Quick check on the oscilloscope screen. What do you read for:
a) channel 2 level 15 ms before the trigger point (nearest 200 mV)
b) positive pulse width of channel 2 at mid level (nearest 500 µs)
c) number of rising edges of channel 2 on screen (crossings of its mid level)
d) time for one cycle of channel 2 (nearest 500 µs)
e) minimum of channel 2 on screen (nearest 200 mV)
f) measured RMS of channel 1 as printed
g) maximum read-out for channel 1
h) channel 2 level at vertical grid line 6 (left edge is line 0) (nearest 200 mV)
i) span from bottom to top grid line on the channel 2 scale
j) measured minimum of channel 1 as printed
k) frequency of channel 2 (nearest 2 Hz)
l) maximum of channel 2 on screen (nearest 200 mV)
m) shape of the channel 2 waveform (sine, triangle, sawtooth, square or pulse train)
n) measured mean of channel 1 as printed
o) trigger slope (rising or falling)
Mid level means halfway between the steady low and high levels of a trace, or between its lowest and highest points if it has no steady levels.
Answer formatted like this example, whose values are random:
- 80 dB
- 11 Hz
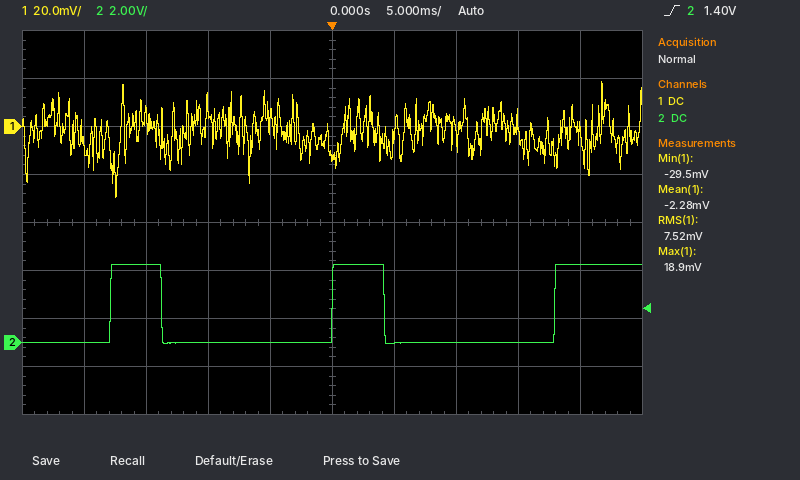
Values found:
- 3.2 V
- 4.0 ms
- 3
- 18.0 ms
- 0.0 V
- 7.52 mV
- 18.9 mV
- 0.0 V
- 16 V
- -29.5 mV
- 56 Hz
- 3.2 V
- pulse train
- -2.28 mV
- rising
